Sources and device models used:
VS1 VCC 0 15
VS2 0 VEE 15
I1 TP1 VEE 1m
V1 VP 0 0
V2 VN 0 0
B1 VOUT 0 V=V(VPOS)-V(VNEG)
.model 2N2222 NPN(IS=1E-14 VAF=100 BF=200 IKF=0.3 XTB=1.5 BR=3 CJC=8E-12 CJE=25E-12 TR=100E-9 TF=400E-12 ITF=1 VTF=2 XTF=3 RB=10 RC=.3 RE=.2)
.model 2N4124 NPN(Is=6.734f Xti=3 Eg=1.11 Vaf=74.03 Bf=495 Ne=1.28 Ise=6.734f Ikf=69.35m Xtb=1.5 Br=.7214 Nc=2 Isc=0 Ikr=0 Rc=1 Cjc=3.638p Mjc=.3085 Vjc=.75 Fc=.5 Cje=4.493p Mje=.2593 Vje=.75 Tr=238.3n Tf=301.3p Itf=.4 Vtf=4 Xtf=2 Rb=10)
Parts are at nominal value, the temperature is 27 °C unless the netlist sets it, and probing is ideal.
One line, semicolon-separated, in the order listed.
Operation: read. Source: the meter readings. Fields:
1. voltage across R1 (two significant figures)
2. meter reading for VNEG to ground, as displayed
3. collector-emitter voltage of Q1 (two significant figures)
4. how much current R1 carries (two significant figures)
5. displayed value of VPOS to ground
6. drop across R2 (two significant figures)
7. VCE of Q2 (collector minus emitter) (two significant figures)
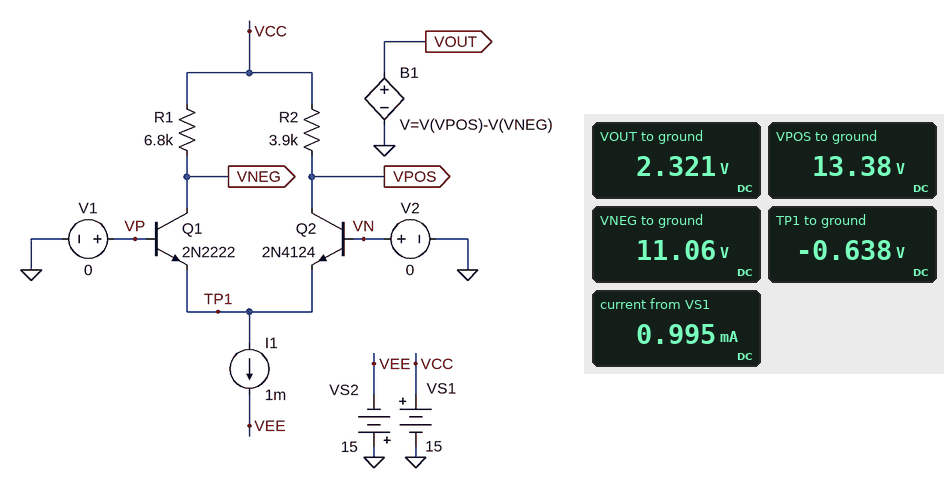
3.9 V; 11.06 V; 12 V; 580 µA; 13.38 V; 1.6 V; 14 V
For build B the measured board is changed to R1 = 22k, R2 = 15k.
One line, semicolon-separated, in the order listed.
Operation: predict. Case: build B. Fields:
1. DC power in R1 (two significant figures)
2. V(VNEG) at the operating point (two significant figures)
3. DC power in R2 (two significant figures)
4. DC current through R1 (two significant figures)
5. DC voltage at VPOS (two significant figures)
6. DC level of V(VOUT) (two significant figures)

7.2 mW; 2.4 V; 2.7 mW; 570 µA; 8.7 V; 6.3 V
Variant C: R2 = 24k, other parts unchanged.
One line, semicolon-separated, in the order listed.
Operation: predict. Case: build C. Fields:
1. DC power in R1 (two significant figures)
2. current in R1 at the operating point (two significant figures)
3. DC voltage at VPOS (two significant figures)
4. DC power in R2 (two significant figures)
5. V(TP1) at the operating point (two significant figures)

2.5 mW; 600 µA; 5.6 V; 3.7 mW; -640 mV
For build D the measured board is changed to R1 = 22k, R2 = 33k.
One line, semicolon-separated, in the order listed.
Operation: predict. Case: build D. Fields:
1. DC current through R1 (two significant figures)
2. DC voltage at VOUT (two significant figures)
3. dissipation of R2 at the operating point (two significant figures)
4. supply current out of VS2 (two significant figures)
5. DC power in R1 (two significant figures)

590 µA; -200 mV; 5.3 mW; 1.0 mA; 7.7 mW
